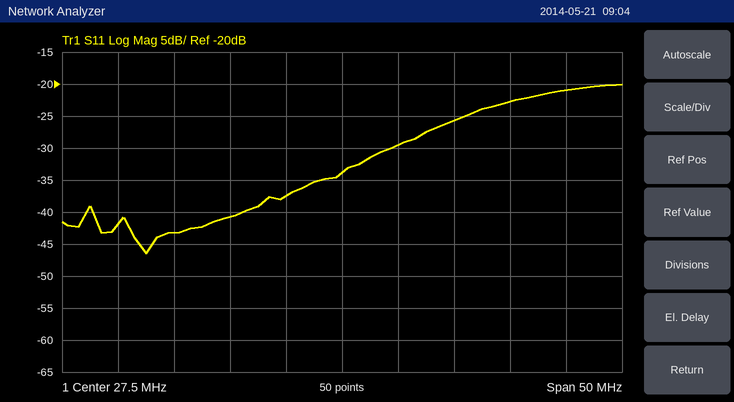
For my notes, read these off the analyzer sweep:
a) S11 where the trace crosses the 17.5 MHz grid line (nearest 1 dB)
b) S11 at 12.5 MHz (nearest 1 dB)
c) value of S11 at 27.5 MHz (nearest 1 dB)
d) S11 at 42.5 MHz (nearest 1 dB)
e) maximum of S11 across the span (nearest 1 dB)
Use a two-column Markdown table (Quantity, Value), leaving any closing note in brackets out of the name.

| Quantity | Value |
|---|---|
| S11 where the trace crosses the 17.5 MHz grid line | -41 dB |
| S11 at 12.5 MHz | -43 dB |
| value of S11 at 27.5 MHz | -34 dB |
| S11 at 42.5 MHz | -23 dB |
| maximum of S11 across the span | -20 dB |
